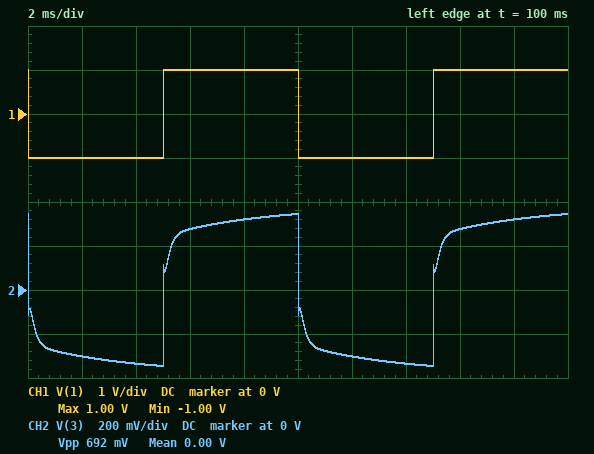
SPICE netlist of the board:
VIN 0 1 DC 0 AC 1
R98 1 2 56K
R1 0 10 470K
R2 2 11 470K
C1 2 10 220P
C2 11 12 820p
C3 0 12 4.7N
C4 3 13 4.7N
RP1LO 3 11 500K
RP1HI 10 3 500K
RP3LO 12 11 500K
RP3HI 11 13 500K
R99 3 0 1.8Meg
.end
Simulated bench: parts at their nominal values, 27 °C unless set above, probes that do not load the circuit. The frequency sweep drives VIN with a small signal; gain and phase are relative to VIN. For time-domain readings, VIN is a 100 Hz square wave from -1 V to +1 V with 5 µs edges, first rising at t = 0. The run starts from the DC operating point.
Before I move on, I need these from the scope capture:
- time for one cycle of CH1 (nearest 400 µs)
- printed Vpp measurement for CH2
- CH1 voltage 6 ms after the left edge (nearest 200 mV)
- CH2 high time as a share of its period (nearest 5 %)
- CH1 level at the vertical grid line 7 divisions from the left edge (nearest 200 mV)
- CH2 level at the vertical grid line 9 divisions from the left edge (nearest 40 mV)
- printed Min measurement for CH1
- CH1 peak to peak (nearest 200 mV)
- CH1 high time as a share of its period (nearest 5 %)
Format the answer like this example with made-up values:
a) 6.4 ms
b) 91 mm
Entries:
a) 10.0 ms
b) 692 mV
c) 1.0 V
d) 50 %
e) -1.0 V
f) 320 mV
g) -1.00 V
h) 2.0 V
i) 50 %
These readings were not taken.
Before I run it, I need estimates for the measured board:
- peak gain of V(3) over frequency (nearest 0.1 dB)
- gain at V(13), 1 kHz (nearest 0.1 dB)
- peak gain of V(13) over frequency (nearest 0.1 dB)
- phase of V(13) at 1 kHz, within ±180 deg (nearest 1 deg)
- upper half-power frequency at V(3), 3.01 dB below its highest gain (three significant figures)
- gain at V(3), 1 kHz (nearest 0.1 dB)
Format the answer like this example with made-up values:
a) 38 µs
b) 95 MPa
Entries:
a) -8.4 dB
b) -13.4 dB
c) -3.3 dB
d) 164 deg
e) 490 Hz
f) -13.1 dB
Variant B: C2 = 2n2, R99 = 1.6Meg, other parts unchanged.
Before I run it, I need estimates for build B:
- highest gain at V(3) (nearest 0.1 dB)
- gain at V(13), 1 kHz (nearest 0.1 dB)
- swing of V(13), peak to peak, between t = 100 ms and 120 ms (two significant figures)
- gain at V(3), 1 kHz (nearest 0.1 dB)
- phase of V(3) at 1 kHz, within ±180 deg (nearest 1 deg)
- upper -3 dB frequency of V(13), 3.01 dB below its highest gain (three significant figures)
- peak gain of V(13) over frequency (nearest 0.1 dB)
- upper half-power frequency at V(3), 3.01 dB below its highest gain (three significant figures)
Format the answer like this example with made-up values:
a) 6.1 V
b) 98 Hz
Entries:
a) -8.6 dB
b) -19.7 dB
c) 930 mV
d) -19.0 dB
e) 163 deg
f) 40.2 Hz
g) -3.4 dB
h) 291 Hz
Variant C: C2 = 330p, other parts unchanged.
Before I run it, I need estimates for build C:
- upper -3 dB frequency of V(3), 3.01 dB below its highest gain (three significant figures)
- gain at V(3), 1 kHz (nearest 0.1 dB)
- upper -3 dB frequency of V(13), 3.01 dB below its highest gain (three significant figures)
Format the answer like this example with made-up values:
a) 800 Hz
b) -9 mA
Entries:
a) 5.56 kHz
b) -10.4 dB
c) 37.6 Hz
